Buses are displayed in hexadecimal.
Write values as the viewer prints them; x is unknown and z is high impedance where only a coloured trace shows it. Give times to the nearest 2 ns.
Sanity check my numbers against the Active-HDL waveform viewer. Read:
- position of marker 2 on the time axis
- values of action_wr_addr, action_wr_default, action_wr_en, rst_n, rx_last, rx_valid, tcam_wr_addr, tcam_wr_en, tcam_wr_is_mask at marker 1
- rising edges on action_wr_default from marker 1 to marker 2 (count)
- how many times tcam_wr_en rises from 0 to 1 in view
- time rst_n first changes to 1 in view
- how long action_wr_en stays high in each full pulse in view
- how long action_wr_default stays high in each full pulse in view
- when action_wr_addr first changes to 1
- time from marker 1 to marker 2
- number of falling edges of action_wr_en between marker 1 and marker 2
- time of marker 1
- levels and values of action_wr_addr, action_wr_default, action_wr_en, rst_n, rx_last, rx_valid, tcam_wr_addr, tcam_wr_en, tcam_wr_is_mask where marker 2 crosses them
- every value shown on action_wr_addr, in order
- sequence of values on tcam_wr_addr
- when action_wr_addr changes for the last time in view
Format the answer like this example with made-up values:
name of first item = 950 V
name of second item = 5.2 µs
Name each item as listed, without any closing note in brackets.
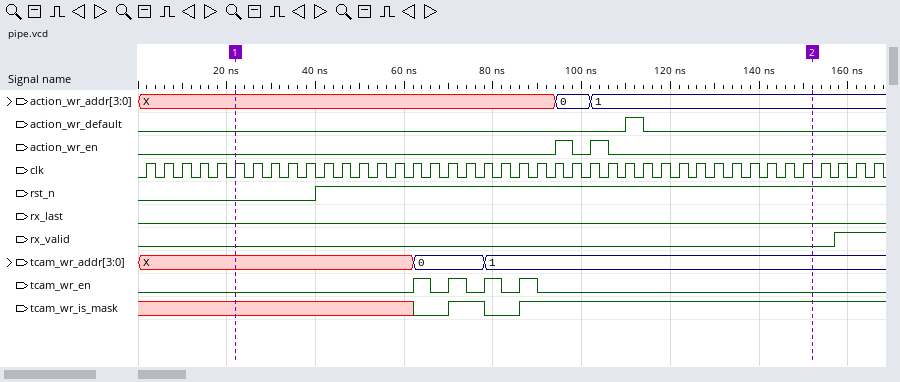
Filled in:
position of marker 2 on the time axis = 152 ns
values of action_wr_addr, action_wr_default, action_wr_en, rst_n, rx_last, rx_valid, tcam_wr_addr, tcam_wr_en, tcam_wr_is_mask at marker 1 = action_wr_addr=X, action_wr_default=0, action_wr_en=0, rst_n=0, rx_last=0, rx_valid=0, tcam_wr_addr=X, tcam_wr_en=0, tcam_wr_is_mask=x
rising edges on action_wr_default from marker 1 to marker 2 = 1
how many times tcam_wr_en rises from 0 to 1 in view = 4
time rst_n first changes to 1 in view = 40 ns
how long action_wr_en stays high in each full pulse in view = 4 ns, 4 ns
how long action_wr_default stays high in each full pulse in view = 4 ns
when action_wr_addr first changes to 1 = 102 ns
time from marker 1 to marker 2 = 130 ns
number of falling edges of action_wr_en between marker 1 and marker 2 = 2
time of marker 1 = 22 ns
levels and values of action_wr_addr, action_wr_default, action_wr_en, rst_n, rx_last, rx_valid, tcam_wr_addr, tcam_wr_en, tcam_wr_is_mask where marker 2 crosses them = action_wr_addr=1, action_wr_default=0, action_wr_en=0, rst_n=1, rx_last=0, rx_valid=0, tcam_wr_addr=1, tcam_wr_en=0, tcam_wr_is_mask=1
every value shown on action_wr_addr, in order = X, 0, 1
sequence of values on tcam_wr_addr = X, 0, 1
when action_wr_addr changes for the last time in view = 102 ns
